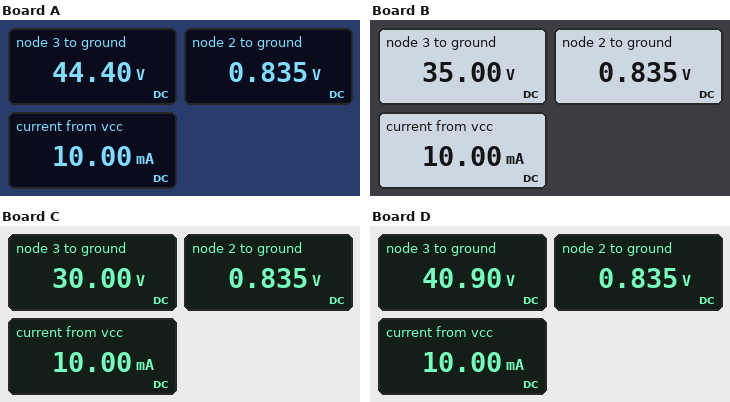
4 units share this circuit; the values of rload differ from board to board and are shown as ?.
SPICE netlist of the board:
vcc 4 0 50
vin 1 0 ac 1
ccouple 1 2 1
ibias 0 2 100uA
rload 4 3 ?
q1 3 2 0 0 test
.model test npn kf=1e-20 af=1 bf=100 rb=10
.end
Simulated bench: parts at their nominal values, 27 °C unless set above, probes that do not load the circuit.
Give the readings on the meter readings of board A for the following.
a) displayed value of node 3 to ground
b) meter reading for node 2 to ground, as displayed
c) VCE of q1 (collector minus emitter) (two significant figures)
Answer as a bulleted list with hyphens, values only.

- 44.40 V
- 0.835 V
- 44 V
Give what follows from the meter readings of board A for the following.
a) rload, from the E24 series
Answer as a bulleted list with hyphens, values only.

- 560 Ω
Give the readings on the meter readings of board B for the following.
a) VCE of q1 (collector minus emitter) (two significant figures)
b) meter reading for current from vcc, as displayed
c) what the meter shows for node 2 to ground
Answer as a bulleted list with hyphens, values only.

- 35 V
- 10.00 mA
- 0.835 V
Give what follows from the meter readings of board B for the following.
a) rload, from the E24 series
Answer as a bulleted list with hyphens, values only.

- 1.5 kΩ
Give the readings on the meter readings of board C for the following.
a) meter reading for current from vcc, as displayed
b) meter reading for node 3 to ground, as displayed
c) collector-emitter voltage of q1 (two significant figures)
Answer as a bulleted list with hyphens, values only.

- 10.00 mA
- 30.00 V
- 30 V
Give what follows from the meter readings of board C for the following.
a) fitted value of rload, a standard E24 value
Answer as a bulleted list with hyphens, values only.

- 2 kΩ
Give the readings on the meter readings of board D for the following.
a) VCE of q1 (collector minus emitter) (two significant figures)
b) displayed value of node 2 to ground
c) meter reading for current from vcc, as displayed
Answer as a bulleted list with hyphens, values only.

- 41 V
- 0.835 V
- 10.00 mA
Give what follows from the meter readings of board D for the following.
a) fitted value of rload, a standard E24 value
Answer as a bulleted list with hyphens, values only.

- 910 Ω
